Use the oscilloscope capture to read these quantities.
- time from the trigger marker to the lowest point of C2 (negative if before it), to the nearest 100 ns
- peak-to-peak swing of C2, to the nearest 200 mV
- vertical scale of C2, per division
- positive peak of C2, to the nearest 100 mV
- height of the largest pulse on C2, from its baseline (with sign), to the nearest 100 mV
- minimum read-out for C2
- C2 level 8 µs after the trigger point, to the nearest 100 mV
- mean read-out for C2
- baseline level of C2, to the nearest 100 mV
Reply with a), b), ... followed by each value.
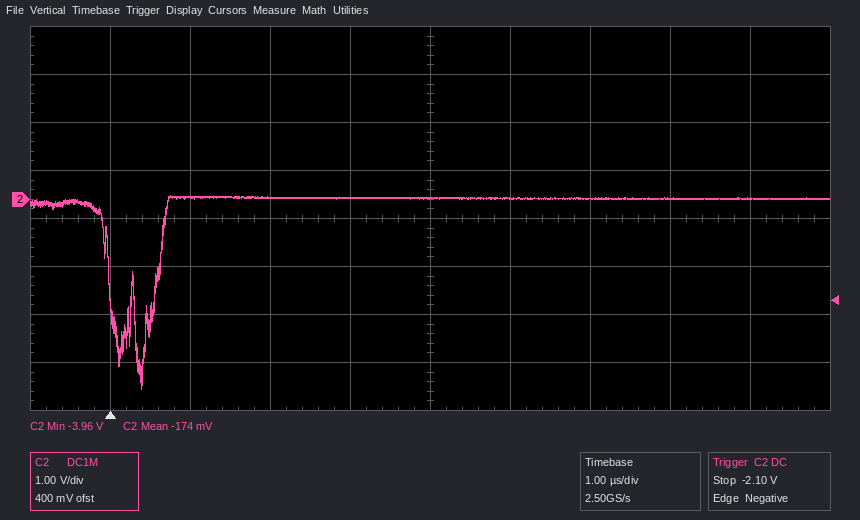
a) +400 ns
b) 4.0 V
c) 1 V
d) 100 mV
e) -4.0 V
f) -3.96 V
g) 0.0 V
h) -174 mV
i) 0.0 V
